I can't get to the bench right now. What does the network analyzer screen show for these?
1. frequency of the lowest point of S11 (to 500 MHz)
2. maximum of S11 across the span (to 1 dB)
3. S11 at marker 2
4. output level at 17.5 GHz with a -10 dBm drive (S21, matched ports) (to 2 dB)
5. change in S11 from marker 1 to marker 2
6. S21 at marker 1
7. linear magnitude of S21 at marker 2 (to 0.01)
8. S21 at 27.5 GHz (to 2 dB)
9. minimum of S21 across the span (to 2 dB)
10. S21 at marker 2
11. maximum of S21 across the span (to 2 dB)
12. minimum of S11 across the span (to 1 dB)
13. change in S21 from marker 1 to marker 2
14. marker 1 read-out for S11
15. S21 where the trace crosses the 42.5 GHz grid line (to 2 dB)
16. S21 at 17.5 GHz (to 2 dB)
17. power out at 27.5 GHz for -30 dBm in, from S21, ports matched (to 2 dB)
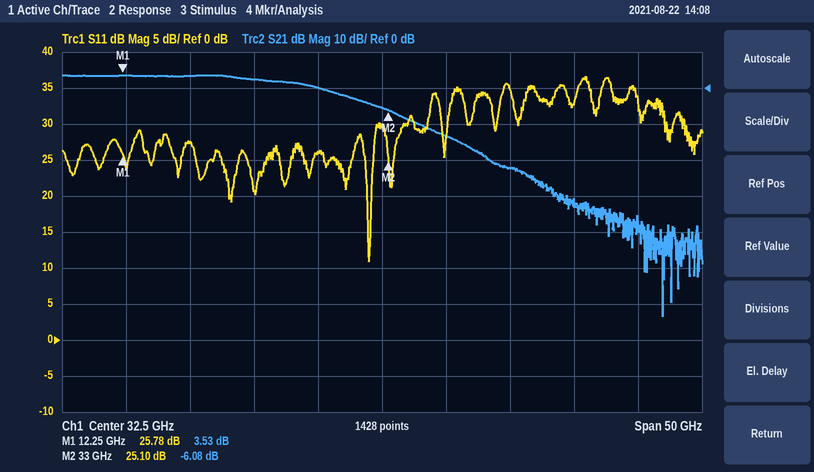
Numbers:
31.5 GHz
37 dB
25.10 dB
-6 dBm
-0.68 dB
3.53 dB
0.50
0 dB
-64 dB
-6.08 dB
4 dB
11 dB
-9.61 dB
25.78 dB
-22 dB
4 dB
-30 dBm
